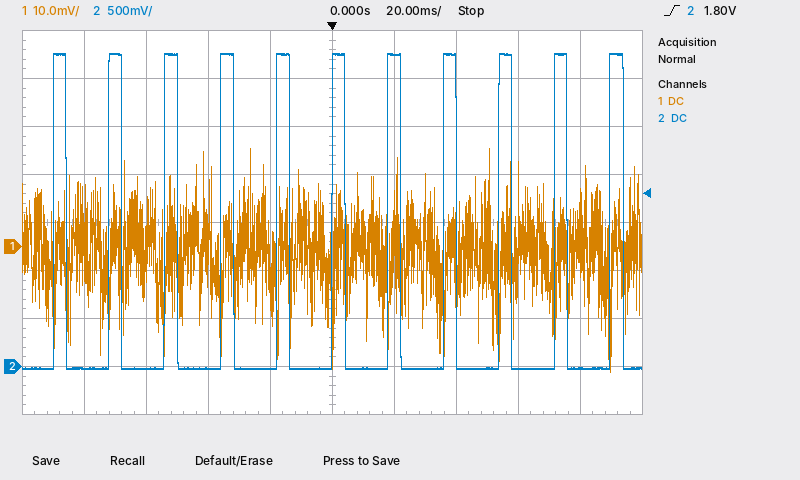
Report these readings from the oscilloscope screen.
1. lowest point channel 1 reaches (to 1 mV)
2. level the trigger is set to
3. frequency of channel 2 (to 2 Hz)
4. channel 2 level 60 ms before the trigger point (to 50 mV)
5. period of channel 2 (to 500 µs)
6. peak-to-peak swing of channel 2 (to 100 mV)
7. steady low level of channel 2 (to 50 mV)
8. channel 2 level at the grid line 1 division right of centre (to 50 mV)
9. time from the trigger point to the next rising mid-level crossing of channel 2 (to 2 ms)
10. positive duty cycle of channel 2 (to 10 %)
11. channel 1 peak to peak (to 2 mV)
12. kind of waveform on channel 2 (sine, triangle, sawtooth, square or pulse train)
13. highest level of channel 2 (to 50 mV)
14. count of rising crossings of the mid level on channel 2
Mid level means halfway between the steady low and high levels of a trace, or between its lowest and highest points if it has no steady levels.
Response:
-26 mV
1.80 V
56 Hz
0 mV
18.0 ms
3.30 V
0 mV
3.25 V
18 ms
20 %
46 mV
pulse train
3.25 V
11
